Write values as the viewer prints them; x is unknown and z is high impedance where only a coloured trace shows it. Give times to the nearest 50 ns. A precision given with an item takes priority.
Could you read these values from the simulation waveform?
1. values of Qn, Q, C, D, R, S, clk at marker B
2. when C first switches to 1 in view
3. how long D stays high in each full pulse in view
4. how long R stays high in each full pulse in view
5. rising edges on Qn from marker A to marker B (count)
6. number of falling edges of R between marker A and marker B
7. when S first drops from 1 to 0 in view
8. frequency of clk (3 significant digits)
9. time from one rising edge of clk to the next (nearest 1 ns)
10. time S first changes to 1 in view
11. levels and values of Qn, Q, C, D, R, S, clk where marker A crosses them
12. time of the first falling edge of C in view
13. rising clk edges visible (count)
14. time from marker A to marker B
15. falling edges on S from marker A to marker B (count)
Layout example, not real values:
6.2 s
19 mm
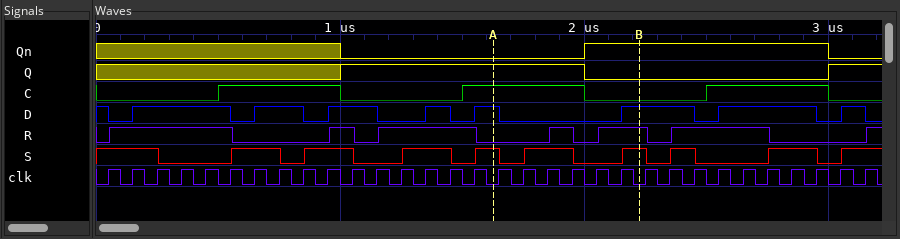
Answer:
Qn=1, Q=0, C=0, D=1, R=1, S=1, clk=0
500 ns
400 ns, 200 ns, 200 ns, 100 ns, 100 ns, 300 ns, 400 ns, 100 ns
500 ns, 100 ns, 400 ns, 100 ns, 200 ns, 400 ns
1
1
250 ns
10.0 MHz
100 ns
550 ns
Qn=0, Q=1, C=1, D=1, R=0, S=1, clk=0
1000 ns
32
600 ns
2
